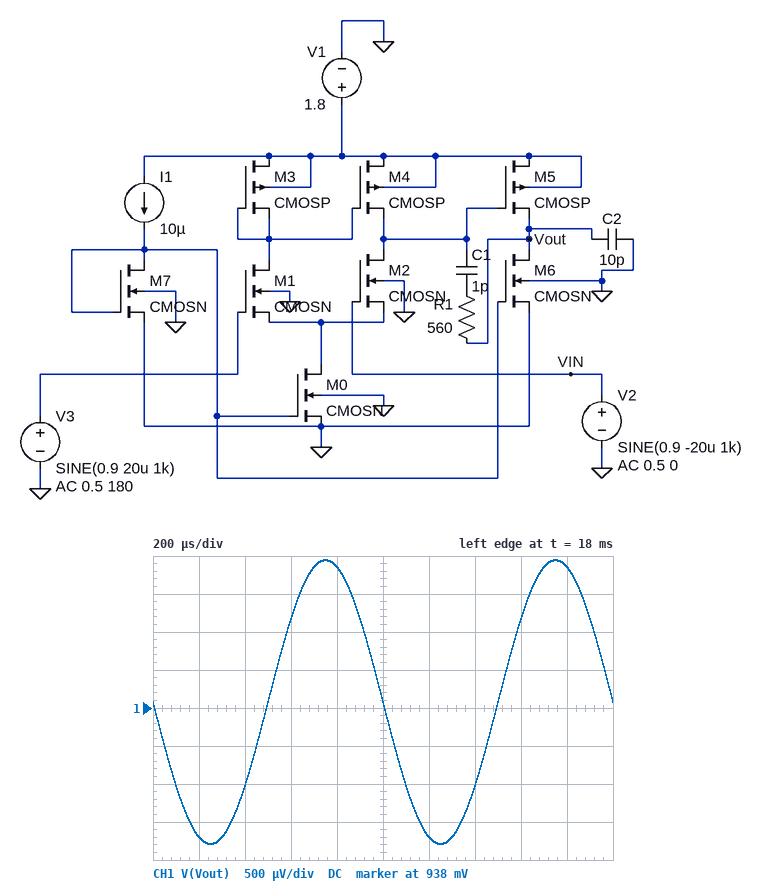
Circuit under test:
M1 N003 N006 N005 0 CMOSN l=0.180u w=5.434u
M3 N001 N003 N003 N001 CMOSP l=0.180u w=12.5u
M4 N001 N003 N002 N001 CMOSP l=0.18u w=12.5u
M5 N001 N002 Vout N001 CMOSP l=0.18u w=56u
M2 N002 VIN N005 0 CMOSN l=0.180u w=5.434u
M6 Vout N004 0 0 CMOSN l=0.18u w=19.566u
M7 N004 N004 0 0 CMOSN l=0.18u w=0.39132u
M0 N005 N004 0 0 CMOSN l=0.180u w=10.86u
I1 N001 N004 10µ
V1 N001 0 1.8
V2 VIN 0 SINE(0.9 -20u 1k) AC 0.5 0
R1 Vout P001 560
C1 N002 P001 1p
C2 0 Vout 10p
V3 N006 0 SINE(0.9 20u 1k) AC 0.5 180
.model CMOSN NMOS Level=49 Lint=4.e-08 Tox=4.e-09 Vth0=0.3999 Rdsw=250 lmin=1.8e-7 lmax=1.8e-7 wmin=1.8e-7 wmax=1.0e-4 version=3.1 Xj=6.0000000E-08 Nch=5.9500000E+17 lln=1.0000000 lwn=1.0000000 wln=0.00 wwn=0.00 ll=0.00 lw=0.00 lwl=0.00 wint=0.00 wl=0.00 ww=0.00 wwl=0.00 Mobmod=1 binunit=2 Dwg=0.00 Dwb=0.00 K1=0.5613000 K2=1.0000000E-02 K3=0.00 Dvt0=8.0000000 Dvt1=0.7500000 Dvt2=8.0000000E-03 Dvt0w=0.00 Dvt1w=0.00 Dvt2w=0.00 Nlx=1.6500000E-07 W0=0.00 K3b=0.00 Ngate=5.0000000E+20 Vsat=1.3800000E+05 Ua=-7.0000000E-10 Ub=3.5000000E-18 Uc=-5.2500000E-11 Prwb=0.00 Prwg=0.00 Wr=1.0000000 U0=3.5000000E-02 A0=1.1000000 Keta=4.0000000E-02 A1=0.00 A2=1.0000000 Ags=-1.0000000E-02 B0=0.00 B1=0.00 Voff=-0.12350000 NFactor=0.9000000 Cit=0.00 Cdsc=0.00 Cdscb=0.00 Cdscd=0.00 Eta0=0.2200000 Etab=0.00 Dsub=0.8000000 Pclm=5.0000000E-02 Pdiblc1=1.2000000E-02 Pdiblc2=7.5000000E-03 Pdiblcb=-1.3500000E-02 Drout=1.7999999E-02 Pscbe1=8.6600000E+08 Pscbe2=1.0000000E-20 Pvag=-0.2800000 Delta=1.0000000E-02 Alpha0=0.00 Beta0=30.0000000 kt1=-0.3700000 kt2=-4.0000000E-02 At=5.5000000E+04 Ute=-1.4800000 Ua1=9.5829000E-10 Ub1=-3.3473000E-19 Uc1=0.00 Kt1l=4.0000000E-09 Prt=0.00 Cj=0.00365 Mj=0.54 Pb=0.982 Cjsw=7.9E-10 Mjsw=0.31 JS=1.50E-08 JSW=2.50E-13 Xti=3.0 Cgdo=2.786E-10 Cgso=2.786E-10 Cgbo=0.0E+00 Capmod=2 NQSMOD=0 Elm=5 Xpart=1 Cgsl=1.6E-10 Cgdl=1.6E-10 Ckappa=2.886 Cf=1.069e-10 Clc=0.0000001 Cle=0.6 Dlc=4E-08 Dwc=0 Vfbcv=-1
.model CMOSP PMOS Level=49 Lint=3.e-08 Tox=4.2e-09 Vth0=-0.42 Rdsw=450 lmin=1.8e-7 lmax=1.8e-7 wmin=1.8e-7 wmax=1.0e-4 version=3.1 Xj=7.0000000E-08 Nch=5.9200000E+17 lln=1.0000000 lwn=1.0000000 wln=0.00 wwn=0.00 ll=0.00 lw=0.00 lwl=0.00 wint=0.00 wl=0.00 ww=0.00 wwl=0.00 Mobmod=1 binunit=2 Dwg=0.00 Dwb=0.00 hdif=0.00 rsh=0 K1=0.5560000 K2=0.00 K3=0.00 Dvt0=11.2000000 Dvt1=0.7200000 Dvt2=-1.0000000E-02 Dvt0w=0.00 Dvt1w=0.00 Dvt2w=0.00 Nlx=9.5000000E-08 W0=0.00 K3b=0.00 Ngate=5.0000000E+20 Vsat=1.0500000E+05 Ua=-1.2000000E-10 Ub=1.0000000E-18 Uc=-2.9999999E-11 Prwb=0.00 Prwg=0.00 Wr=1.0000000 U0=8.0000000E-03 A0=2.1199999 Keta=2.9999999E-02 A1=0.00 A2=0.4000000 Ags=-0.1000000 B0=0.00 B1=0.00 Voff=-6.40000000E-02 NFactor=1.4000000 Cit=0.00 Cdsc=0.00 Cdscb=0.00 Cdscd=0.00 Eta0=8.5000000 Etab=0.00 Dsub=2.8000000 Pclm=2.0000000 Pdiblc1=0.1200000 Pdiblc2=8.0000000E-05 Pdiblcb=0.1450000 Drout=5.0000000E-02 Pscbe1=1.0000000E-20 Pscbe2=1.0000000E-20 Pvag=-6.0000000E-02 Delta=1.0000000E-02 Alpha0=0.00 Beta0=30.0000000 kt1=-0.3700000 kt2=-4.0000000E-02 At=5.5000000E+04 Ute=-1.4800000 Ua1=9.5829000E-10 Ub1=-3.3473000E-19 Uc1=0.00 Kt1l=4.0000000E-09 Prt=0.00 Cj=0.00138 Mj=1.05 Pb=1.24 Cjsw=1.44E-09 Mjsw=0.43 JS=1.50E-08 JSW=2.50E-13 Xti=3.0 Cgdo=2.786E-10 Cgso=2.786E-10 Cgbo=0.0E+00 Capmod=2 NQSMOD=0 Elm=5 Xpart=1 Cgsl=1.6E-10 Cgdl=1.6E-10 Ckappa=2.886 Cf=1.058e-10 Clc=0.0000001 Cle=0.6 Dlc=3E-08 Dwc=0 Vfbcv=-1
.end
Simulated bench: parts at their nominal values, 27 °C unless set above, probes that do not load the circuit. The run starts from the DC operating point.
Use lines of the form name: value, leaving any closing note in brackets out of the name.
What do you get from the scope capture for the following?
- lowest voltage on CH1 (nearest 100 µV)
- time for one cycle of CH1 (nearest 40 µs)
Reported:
lowest voltage on CH1: 936.2 mV
time for one cycle of CH1: 1.00 ms
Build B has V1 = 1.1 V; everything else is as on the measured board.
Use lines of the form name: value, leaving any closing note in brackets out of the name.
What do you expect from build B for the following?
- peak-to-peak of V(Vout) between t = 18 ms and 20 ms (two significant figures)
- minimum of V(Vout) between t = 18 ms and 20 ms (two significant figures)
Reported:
peak-to-peak of V(Vout) between t = 18 ms and 20 ms: 3.1 mV
minimum of V(Vout) between t = 18 ms and 20 ms: 590 mV
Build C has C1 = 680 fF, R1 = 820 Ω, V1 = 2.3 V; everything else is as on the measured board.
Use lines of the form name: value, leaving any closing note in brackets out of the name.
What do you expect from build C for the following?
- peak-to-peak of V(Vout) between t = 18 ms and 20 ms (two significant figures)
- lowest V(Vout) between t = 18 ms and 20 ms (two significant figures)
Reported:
peak-to-peak of V(Vout) between t = 18 ms and 20 ms: 4.1 mV
lowest V(Vout) between t = 18 ms and 20 ms: 1.2 V
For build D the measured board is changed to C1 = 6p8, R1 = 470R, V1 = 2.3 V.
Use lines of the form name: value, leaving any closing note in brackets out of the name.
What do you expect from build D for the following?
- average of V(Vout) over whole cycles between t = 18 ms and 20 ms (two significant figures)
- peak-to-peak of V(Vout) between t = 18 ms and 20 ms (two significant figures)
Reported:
average of V(Vout) over whole cycles between t = 18 ms and 20 ms: 1.2 V
peak-to-peak of V(Vout) between t = 18 ms and 20 ms: 4.1 mV
